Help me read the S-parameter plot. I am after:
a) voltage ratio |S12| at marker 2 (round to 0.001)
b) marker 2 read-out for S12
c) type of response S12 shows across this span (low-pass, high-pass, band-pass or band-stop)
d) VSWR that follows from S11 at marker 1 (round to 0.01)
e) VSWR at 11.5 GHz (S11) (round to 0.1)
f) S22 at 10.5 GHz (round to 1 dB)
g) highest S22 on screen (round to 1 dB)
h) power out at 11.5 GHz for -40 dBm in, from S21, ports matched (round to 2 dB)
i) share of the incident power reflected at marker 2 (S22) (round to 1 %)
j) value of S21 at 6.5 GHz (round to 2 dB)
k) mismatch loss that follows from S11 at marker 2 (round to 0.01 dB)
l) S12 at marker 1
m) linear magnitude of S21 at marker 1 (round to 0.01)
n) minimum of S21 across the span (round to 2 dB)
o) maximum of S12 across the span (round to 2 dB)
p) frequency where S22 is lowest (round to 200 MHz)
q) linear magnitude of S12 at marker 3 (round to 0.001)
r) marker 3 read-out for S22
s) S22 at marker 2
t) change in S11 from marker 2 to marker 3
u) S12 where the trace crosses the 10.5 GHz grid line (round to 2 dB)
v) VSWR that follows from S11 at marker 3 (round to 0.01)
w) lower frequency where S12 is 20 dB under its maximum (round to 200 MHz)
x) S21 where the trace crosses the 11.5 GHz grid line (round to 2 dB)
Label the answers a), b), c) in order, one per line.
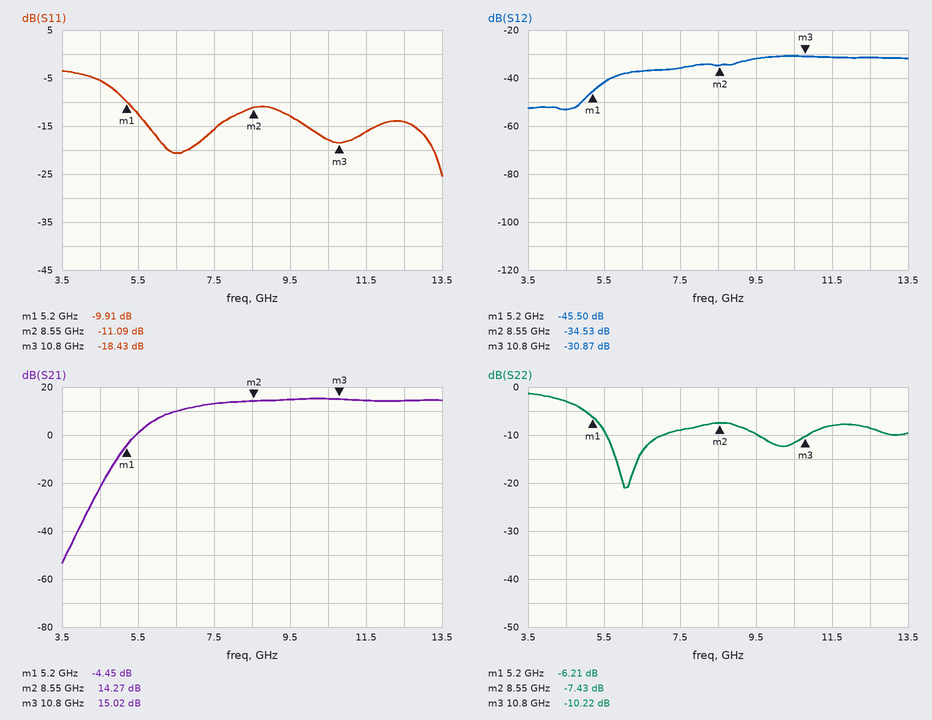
a) 0.019
b) -34.53 dB
c) high-pass
d) 1.94
e) 1.4
f) -12 dB
g) -1 dB
h) -26 dBm
i) 18 %
j) 10 dB
k) 0.35 dB
l) -45.50 dB
m) 0.60
n) -54 dB
o) -30 dB
p) 6.0 GHz
q) 0.029
r) -10.22 dB
s) -7.43 dB
t) -7.34 dB
u) -30 dB
v) 1.27
w) 4.8 GHz
x) 14 dB
